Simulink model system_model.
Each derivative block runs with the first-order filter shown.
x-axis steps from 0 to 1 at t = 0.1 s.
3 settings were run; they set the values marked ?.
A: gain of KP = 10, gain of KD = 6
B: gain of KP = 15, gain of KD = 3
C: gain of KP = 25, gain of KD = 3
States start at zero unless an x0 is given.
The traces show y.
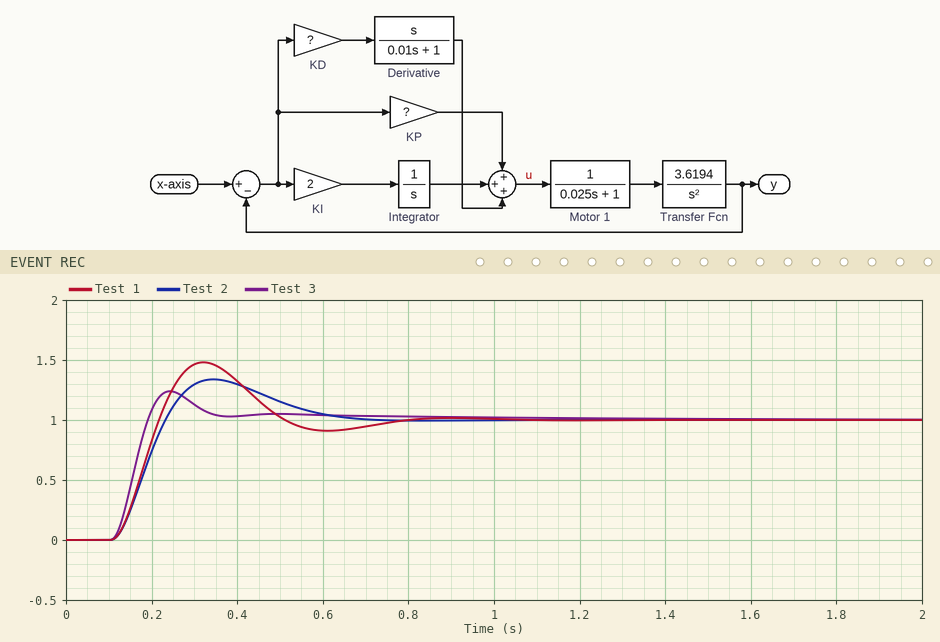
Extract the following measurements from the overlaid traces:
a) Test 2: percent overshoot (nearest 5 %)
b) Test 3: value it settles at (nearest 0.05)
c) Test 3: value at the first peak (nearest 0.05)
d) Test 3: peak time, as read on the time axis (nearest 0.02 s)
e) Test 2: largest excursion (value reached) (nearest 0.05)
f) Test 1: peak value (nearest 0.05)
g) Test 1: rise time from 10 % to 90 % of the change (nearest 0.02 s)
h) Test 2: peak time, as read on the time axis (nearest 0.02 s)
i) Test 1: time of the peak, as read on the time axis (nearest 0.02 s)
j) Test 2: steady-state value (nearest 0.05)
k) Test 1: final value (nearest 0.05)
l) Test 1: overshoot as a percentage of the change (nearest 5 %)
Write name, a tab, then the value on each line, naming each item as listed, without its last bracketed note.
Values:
Test 2: percent overshoot	35 %
Test 3: value it settles at	1.00
Test 3: value at the first peak	1.25
Test 3: peak time, as read on the time axis	0.24 s
Test 2: largest excursion (value reached)	1.35
Test 1: peak value	1.50
Test 1: rise time from 10 % to 90 % of the change	0.08 s
Test 2: peak time, as read on the time axis	0.34 s
Test 1: time of the peak, as read on the time axis	0.32 s
Test 2: steady-state value	1.00
Test 1: final value	1.00
Test 1: overshoot as a percentage of the change	50 %
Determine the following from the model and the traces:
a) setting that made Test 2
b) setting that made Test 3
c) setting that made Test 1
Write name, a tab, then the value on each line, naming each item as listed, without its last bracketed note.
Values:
setting that made Test 2	B
setting that made Test 3	A
setting that made Test 1	C
